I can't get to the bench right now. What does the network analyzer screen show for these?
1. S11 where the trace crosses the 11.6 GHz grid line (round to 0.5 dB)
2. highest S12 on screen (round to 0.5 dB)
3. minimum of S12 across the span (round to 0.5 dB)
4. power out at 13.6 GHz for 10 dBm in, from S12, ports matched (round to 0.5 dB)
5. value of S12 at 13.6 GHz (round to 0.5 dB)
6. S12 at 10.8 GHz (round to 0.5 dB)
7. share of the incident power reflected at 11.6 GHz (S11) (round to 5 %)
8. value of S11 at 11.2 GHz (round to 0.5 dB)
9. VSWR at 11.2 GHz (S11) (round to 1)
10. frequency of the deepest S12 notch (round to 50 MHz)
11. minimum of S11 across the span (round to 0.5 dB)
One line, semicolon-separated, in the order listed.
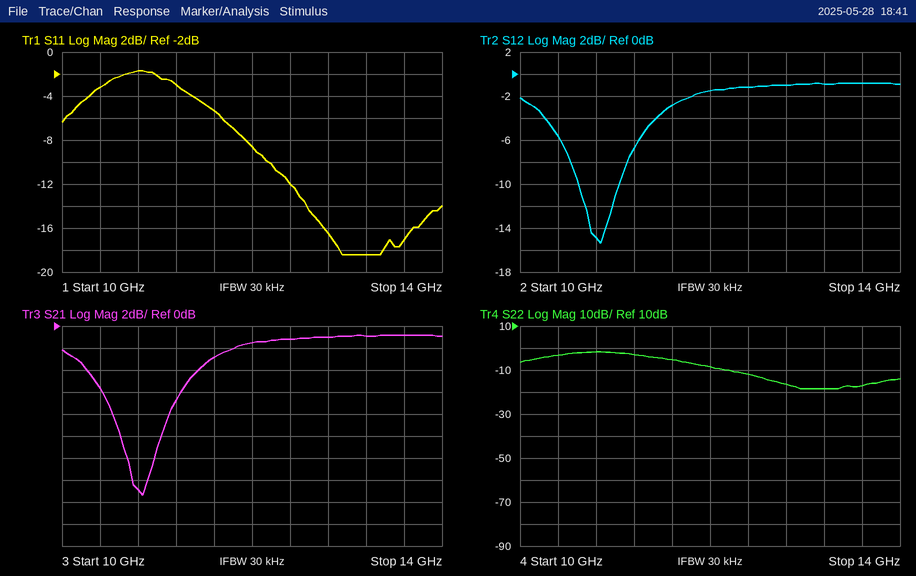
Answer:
-5.5 dB; -1.0 dB; -15.5 dB; 9.0 dBm; -1.0 dB; -15.0 dB; 30 %; -3.0 dB; 6; 10.85 GHz; -18.5 dB
